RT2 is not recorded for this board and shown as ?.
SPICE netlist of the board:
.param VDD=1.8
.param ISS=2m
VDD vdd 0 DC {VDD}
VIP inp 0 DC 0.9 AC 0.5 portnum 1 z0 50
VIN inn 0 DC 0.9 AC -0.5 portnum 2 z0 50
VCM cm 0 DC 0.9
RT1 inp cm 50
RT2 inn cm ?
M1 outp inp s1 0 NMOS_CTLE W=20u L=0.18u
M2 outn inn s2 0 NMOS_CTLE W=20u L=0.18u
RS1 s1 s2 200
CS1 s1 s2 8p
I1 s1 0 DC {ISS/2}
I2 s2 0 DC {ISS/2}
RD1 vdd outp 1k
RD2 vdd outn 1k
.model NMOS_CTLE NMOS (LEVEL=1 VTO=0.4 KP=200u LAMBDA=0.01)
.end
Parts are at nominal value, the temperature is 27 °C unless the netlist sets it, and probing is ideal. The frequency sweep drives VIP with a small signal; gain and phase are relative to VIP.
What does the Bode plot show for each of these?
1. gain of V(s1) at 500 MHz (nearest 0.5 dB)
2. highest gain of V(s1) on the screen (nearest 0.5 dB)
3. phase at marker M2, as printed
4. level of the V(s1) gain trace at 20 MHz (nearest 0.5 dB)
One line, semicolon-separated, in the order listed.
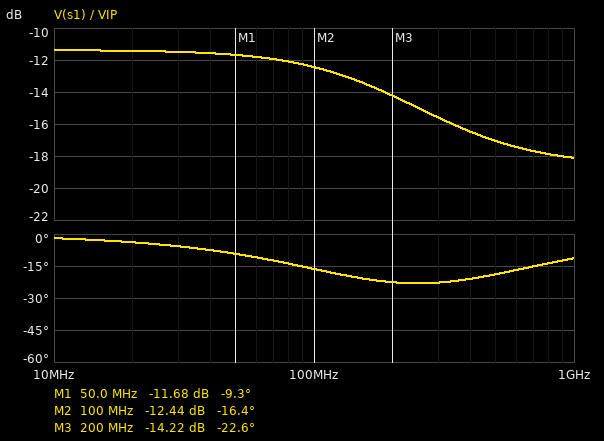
-17.0 dB; -11.5 dB; -16.4 deg; -11.5 dB
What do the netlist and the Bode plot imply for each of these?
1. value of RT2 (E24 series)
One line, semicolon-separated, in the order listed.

56 Ω
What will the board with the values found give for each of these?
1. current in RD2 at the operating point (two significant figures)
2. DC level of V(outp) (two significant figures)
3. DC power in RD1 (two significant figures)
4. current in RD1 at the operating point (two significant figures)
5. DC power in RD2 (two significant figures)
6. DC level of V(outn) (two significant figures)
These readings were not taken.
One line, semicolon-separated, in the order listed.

1.0 mA; 800 mV; 1.0 mW; 1.0 mA; 1.0 mW; 800 mV
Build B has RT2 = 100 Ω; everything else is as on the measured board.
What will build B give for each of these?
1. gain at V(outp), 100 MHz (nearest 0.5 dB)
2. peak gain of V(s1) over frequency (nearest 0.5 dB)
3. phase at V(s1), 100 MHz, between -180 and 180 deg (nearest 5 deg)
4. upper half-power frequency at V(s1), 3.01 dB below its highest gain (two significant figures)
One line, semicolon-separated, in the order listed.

6.0 dB; -12.0 dB; -20 deg; 190 MHz
